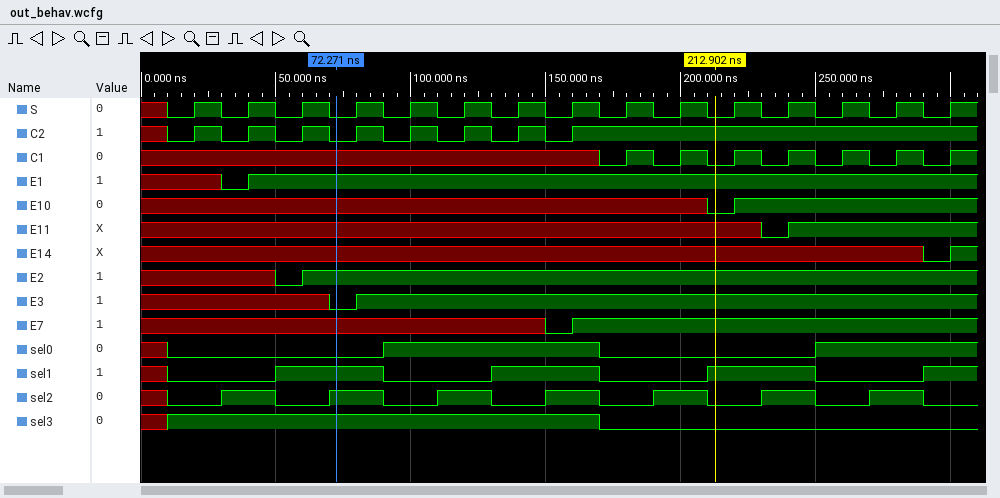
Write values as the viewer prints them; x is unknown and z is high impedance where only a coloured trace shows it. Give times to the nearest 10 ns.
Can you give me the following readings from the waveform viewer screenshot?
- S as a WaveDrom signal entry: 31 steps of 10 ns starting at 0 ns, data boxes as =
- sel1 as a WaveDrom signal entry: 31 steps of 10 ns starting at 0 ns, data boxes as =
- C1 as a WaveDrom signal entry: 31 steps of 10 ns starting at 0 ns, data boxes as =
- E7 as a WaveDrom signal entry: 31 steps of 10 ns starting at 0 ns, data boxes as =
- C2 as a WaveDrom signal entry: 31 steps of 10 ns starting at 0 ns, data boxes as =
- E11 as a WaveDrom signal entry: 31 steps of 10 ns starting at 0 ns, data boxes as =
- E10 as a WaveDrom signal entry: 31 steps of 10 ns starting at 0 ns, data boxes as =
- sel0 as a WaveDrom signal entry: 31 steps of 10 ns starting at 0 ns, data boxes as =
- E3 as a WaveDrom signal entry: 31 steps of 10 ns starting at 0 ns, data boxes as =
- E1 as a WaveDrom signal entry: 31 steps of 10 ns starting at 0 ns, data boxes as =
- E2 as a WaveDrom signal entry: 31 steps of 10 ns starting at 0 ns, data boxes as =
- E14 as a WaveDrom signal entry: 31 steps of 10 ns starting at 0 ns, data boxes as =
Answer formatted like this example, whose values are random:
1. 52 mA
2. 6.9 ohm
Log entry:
1. {name: 'S', wave: 'x010101010101010101010101010101'}
2. {name: 'sel1', wave: 'x0...1...0...1...0...1...0...1.'}
3. {name: 'C1', wave: 'x................01010101010101'}
4. {name: 'E7', wave: 'x..............01..............'}
5. {name: 'C2', wave: 'x0101010101010101..............'}
6. {name: 'E11', wave: 'x......................01......'}
7. {name: 'E10', wave: 'x....................01........'}
8. {name: 'sel0', wave: 'x0.......1.......0.......1.....'}
9. {name: 'E3', wave: 'x......01......................'}
10. {name: 'E1', wave: 'x..01..........................'}
11. {name: 'E2', wave: 'x....01........................'}
12. {name: 'E14', wave: 'x............................01'}
